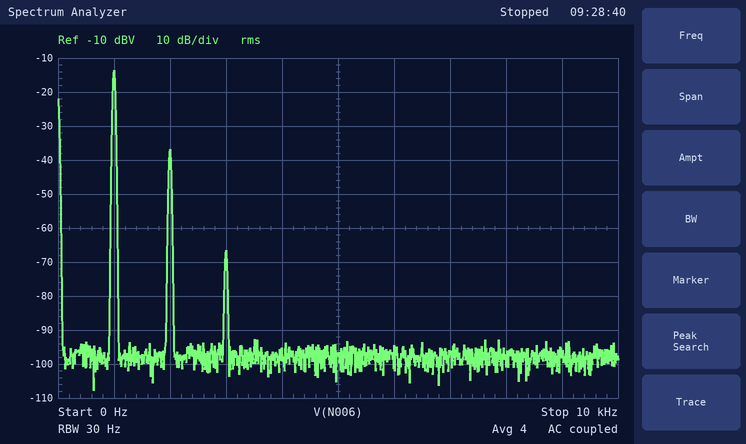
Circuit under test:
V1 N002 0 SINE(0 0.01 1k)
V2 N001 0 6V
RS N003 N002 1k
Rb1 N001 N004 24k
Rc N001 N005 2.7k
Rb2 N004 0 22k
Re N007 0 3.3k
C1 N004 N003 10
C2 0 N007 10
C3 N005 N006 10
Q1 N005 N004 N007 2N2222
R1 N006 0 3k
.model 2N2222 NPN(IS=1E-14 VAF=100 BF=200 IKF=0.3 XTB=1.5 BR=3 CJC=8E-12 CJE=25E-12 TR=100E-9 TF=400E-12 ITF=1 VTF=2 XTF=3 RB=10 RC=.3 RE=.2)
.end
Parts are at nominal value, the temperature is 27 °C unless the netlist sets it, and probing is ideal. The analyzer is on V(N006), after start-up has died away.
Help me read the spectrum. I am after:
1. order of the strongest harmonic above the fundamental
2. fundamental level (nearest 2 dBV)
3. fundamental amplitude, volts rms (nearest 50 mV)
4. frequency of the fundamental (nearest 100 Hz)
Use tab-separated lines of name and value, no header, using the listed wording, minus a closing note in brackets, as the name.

order of the strongest harmonic above the fundamental	2
fundamental level	-14 dBV
fundamental amplitude, volts rms	200 mV
frequency of the fundamental	1.0 kHz
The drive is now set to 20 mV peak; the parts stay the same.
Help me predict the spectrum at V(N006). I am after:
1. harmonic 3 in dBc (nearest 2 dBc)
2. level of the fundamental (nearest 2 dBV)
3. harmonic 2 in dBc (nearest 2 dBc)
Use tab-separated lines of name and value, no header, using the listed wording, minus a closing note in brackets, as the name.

harmonic 3 in dBc	-42 dBc
level of the fundamental	-8 dBV
harmonic 2 in dBc	-18 dBc
